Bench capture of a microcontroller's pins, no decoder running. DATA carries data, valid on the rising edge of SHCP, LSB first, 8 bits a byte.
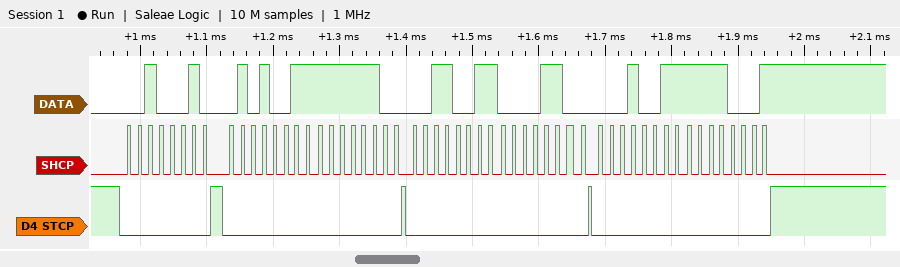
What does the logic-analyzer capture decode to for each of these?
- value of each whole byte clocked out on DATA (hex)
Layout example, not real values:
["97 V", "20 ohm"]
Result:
["44 CA 3F CC 30 C8 8F"]
